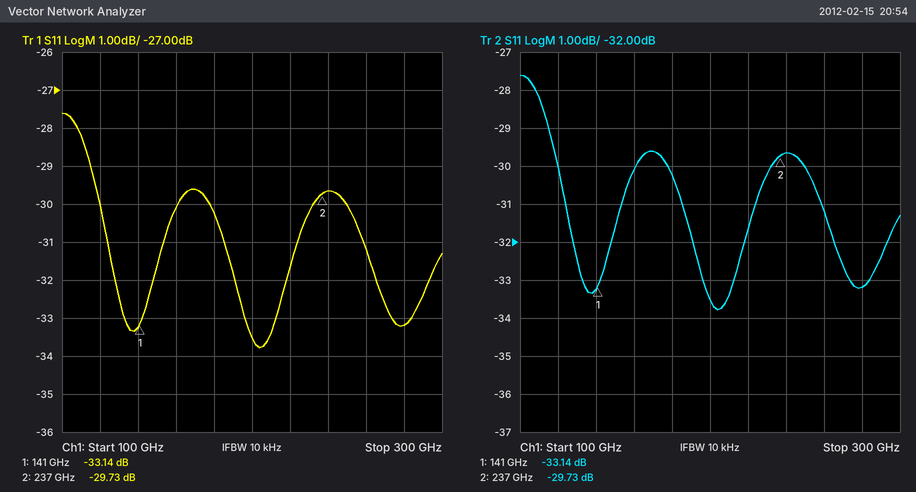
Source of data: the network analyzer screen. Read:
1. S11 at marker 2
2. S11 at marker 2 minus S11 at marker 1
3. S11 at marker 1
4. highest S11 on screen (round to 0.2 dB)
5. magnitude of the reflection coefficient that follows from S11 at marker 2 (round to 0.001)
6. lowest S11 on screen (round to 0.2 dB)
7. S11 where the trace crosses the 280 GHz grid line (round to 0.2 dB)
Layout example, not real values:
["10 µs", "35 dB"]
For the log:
["-29.73 dB", "3.41 dB", "-33.14 dB", "-27.6 dB", "0.033", "-33.8 dB", "-33.2 dB"]
